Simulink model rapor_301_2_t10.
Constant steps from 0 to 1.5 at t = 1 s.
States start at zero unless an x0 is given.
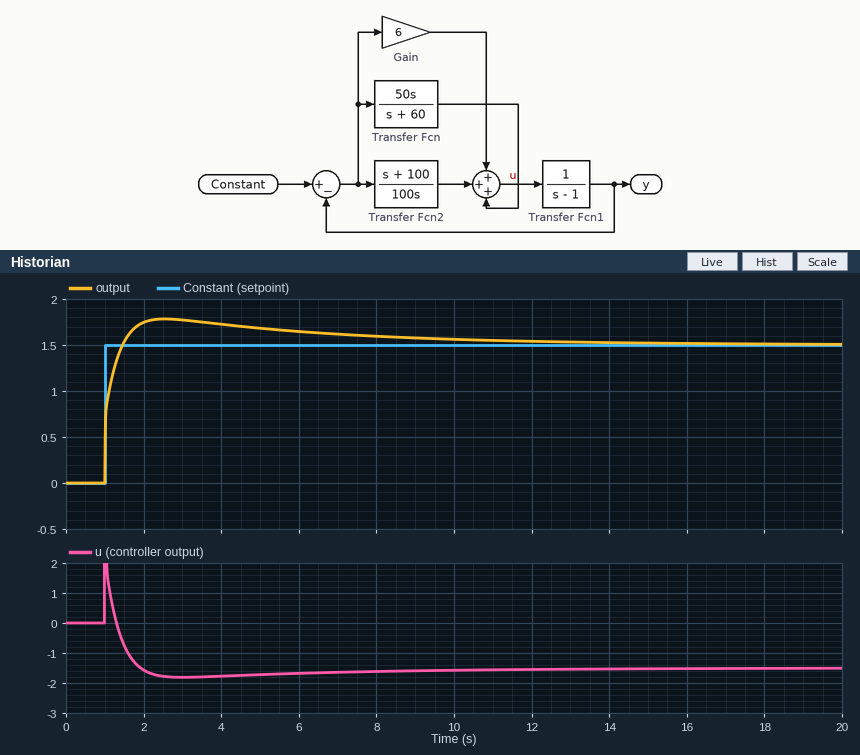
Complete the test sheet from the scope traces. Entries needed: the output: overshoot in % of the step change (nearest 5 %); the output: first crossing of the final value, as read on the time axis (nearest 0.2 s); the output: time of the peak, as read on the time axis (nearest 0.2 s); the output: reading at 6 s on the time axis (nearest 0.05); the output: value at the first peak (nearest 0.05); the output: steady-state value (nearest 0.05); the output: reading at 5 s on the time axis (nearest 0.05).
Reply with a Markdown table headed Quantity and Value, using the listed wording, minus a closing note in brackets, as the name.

| Quantity | Value |
|---|---|
| the output: overshoot in % of the step change | 20 % |
| the output: first crossing of the final value, as read on the time axis | 1.4 s |
| the output: time of the peak, as read on the time axis | 2.6 s |
| the output: reading at 6 s on the time axis | 1.65 |
| the output: value at the first peak | 1.80 |
| the output: steady-state value | 1.50 |
| the output: reading at 5 s on the time axis | 1.70 |
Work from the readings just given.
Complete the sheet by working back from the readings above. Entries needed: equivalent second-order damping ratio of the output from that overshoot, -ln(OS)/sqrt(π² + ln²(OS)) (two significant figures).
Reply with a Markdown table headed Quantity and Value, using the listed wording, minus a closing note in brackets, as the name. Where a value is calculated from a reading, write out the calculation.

| Quantity | Value |
|---|---|
| equivalent second-order damping ratio of the output from that overshoot, -ln(OS)/sqrt(π² + ln²(OS)) | ln(0.2) = -1.609; 1.609 / sqrt(9.870 + 2.590) = 0.46 |
